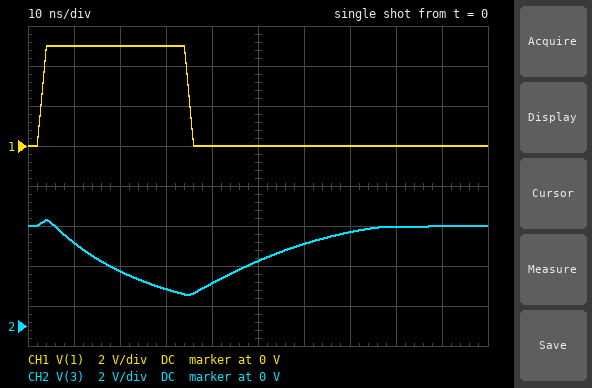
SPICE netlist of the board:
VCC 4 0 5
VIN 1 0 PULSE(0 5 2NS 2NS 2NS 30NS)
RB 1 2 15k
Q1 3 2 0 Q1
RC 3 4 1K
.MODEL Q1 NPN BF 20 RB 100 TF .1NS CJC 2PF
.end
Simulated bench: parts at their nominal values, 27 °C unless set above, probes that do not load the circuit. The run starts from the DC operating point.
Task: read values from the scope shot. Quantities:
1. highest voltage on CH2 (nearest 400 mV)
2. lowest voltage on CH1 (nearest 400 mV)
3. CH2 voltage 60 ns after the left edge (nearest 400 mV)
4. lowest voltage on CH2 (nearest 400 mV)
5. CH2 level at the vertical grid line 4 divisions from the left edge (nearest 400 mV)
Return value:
5.2 V
0 V
4.0 V
1.6 V
2.0 V
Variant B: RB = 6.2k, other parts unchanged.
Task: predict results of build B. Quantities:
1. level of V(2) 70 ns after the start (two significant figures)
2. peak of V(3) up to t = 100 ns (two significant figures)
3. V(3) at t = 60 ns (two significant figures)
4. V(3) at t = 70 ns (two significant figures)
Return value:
660 mV
5.4 V
3.8 V
4.9 V
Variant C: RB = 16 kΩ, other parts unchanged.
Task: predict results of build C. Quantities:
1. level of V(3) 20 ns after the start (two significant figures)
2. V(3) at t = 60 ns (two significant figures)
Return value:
2.9 V
4.2 V
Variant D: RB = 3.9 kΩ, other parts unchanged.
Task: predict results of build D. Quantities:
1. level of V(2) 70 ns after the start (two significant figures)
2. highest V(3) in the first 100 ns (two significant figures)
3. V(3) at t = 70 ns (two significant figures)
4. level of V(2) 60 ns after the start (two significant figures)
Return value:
130 mV
5.4 V
5.0 V
710 mV
